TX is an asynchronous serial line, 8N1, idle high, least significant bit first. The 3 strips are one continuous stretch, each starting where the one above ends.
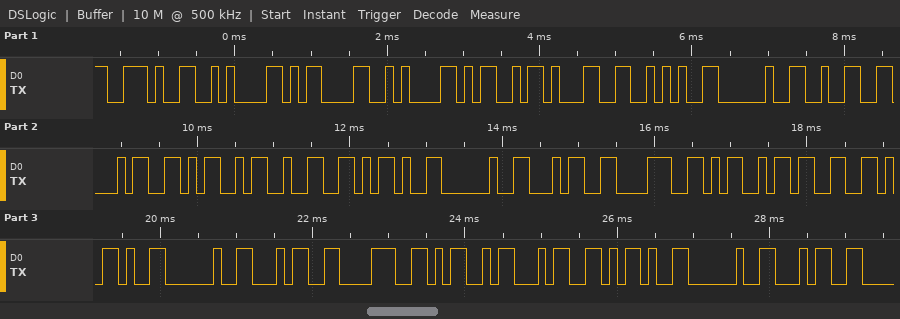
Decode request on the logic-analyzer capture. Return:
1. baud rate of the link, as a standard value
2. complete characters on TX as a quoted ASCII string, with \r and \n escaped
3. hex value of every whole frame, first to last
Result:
9600 baud
".\n\r\nM1* 24M2- 48M3- 48M4- 4"
2E 0A 0D 0A 4D 31 2A 20 32 34 4D 32 2D 20 34 38 4D 33 2D 20 34 38 4D 34 2D 20 34
